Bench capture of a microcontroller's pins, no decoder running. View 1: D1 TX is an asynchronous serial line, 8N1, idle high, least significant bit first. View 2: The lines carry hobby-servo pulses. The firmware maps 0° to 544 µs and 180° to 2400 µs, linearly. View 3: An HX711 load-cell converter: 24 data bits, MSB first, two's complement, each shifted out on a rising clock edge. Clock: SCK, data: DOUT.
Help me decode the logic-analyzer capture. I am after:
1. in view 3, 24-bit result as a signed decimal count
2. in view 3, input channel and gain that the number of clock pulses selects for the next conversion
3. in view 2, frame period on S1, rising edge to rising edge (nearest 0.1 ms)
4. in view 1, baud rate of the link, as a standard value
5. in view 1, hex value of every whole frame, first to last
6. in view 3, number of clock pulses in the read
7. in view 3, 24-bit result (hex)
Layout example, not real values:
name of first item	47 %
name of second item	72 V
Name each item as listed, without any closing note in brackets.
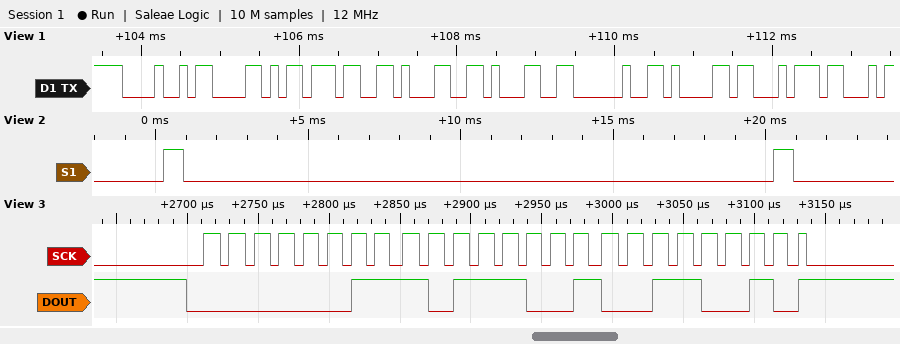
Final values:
in view 3, 24-bit result as a signed decimal count	244018
in view 3, input channel and gain that the number of clock pulses selects for the next conversion	channel A, gain 128
in view 2, frame period on S1, rising edge to rising edge	20.0 ms
in view 1, baud rate of the link, as a standard value	9600 baud
in view 1, hex value of every whole frame, first to last	48 58 37 31 31 20 61 74
in view 3, number of clock pulses in the read	25
in view 3, 24-bit result	0x03B932
